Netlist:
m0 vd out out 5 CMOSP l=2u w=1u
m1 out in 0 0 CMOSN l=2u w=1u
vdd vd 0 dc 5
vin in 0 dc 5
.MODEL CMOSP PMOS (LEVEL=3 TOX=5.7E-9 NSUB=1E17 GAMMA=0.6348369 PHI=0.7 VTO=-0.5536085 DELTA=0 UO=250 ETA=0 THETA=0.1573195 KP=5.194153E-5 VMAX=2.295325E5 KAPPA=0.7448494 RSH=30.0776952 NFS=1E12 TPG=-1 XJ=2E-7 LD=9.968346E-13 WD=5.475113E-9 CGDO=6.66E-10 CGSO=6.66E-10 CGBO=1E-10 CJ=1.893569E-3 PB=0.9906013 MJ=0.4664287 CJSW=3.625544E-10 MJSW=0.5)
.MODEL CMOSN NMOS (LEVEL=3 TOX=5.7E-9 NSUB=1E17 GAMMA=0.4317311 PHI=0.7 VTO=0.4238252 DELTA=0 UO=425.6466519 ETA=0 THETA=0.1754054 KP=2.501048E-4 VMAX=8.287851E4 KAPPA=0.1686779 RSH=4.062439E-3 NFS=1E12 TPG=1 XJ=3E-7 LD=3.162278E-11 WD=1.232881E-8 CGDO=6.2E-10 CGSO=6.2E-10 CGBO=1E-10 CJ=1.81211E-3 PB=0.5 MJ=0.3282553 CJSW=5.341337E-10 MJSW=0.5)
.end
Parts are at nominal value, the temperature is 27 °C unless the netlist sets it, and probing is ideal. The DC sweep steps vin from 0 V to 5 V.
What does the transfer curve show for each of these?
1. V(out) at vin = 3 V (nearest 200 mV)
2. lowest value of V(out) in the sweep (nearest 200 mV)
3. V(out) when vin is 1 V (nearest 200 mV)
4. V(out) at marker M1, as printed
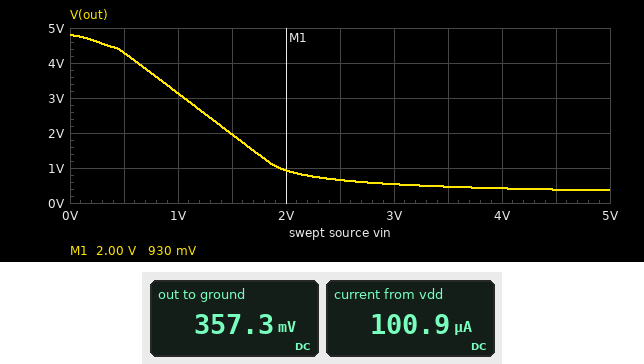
600 mV
400 mV
3.2 V
930 mV
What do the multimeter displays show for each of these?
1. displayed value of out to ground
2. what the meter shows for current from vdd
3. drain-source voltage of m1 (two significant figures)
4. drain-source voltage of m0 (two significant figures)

357.3 mV
100.9 µA
360 mV
4.6 V
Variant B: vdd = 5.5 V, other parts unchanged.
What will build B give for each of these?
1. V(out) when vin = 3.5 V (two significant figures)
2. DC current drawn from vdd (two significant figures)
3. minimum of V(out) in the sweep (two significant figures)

560 mV
120 µA
420 mV
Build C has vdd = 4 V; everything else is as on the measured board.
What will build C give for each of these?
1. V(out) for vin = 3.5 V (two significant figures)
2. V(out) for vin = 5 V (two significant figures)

310 mV
240 mV
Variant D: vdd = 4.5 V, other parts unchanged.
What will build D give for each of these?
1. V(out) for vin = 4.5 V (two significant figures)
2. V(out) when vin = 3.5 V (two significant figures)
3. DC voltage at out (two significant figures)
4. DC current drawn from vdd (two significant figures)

320 mV
380 mV
300 mV
85 µA
